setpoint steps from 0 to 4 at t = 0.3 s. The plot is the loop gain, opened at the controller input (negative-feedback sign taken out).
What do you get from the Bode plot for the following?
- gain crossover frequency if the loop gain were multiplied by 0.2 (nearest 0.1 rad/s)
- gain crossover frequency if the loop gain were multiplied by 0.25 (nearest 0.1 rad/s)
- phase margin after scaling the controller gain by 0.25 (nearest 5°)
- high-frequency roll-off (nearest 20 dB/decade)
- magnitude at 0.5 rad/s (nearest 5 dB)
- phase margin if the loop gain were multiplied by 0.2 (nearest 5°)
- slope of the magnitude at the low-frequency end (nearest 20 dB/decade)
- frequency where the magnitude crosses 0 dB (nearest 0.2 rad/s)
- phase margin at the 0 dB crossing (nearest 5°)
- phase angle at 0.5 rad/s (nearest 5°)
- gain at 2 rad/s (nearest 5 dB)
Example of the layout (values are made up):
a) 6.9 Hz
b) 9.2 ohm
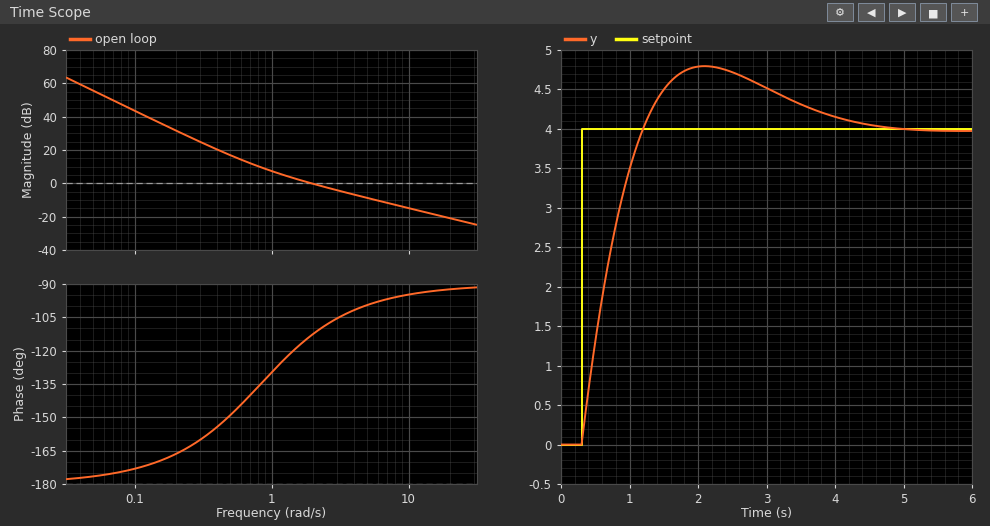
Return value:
a) 0.6 rad/s
b) 0.7 rad/s
c) 40°
d) -20 dB/decade
e) 15 dB
f) 35°
g) -40 dB/decade
h) 2.0 rad/s
i) 65°
j) -150°
k) 0 dB
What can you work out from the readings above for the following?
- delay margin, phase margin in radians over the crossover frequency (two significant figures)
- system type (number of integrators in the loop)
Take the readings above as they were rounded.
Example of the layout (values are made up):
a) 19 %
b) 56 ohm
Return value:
a) 0.57 s
b) 2
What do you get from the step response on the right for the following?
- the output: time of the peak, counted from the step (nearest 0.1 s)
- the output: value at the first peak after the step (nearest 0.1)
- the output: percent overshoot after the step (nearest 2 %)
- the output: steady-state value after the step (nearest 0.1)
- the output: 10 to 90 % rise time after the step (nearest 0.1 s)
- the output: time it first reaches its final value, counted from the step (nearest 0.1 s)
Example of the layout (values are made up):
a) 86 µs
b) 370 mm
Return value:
a) 1.8 s
b) 4.8
c) 20 %
d) 4.0
e) 0.7 s
f) 0.9 s
